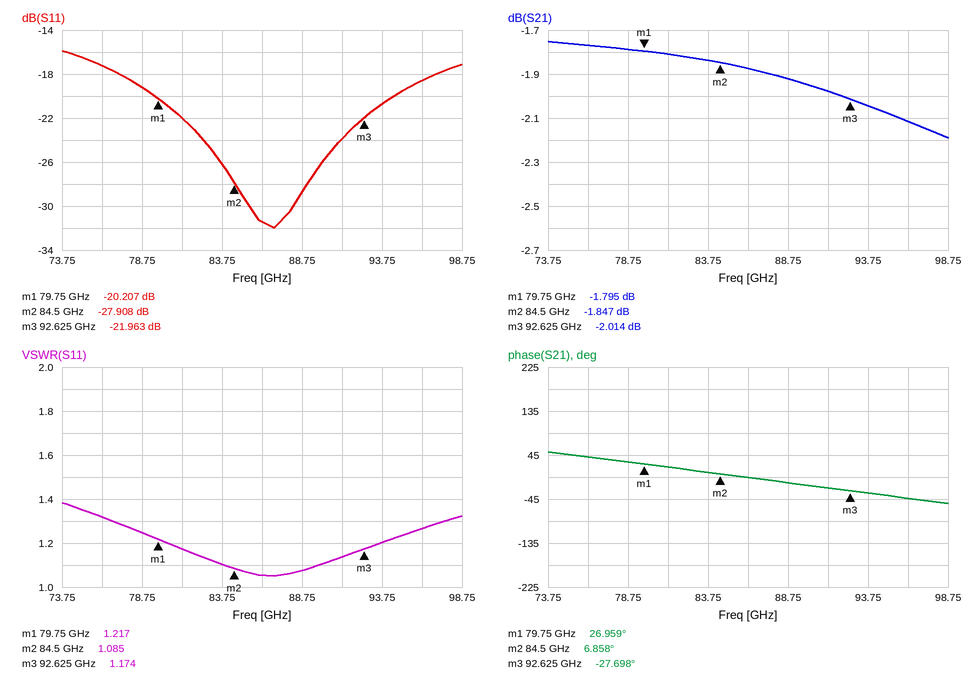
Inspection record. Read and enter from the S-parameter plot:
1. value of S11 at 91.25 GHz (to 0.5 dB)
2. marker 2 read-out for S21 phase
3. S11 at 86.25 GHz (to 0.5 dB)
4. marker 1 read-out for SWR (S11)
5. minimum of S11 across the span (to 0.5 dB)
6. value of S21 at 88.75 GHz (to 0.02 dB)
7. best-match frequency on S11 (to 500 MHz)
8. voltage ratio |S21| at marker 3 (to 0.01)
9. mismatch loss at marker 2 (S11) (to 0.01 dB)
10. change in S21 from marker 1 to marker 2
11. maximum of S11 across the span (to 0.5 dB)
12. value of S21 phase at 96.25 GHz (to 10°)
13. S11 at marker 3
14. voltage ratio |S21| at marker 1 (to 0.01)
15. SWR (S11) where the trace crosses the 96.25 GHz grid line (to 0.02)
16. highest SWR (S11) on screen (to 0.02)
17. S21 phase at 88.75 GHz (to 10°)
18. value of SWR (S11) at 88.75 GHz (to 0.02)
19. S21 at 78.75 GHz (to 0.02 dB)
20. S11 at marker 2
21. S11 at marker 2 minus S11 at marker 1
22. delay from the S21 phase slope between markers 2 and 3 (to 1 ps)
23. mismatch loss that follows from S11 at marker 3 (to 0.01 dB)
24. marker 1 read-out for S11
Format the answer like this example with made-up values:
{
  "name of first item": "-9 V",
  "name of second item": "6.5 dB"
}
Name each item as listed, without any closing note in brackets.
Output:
{
  "value of S11 at 91.25 GHz": "-24.0 dB",
  "marker 2 read-out for S21 phase": "6.858°",
  "S11 at 86.25 GHz": "-31.5 dB",
  "marker 1 read-out for SWR": "1.217",
  "minimum of S11 across the span": "-32.0 dB",
  "value of S21 at 88.75 GHz": "-1.92 dB",
  "best-match frequency on S11": "87.0 GHz",
  "voltage ratio |S21| at marker 3": "0.79",
  "mismatch loss at marker 2 (S11)": "0.01 dB",
  "change in S21 from marker 1 to marker 2": "-0.052 dB",
  "maximum of S11 across the span": "-16.0 dB",
  "value of S21 phase at 96.25 GHz": "-40°",
  "S11 at marker 3": "-21.963 dB",
  "voltage ratio |S21| at marker 1": "0.81",
  "SWR (S11) where the trace crosses the 96.25 GHz grid line": "1.26",
  "highest SWR (S11) on screen": "1.38",
  "S21 phase at 88.75 GHz": "-10°",
  "value of SWR (S11) at 88.75 GHz": "1.08",
  "S21 at 78.75 GHz": "-1.78 dB",
  "S11 at marker 2": "-27.908 dB",
  "S11 at marker 2 minus S11 at marker 1": "-7.701 dB",
  "delay from the S21 phase slope between markers 2 and 3": "12 ps",
  "mismatch loss that follows from S11 at marker 3": "0.03 dB",
  "marker 1 read-out for S11": "-20.207 dB"
}
